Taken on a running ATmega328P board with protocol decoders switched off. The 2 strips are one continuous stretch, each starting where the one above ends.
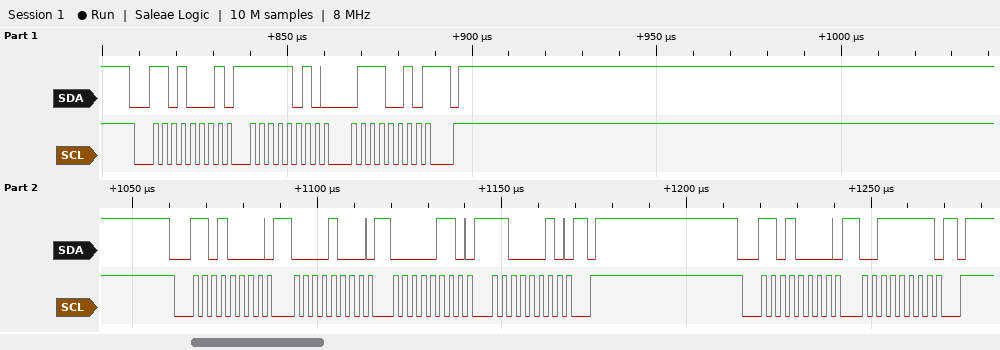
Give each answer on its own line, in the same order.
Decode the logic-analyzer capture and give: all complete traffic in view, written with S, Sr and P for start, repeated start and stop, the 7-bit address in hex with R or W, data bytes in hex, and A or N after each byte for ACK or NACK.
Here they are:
S 68R A FA A 72 N P S 68W A 08 A 06 A C2 A P S 68W A 3F A P
